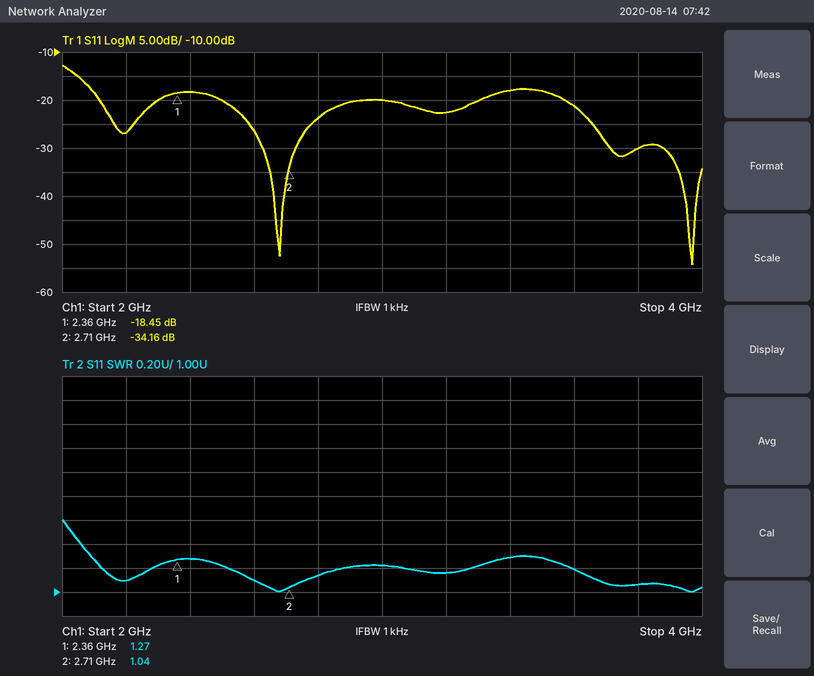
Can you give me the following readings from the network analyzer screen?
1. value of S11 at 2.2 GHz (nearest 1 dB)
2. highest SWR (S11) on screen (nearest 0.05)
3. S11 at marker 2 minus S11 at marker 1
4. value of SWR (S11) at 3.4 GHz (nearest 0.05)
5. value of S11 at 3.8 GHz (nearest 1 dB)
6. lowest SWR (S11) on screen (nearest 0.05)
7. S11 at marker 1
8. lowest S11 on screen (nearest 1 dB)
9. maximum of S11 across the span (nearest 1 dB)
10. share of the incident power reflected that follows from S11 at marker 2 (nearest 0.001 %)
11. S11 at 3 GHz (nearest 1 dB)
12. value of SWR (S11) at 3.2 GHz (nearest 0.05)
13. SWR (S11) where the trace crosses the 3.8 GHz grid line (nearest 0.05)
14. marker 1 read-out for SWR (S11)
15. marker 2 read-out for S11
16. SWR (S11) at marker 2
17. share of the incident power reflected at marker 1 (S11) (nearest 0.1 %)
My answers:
-27 dB
1.60
-15.71 dB
1.30
-30 dB
1.00
-18.45 dB
-54 dB
-13 dB
0.038 %
-20 dB
1.15
1.05
1.27
-34.16 dB
1.04
1.4 %
